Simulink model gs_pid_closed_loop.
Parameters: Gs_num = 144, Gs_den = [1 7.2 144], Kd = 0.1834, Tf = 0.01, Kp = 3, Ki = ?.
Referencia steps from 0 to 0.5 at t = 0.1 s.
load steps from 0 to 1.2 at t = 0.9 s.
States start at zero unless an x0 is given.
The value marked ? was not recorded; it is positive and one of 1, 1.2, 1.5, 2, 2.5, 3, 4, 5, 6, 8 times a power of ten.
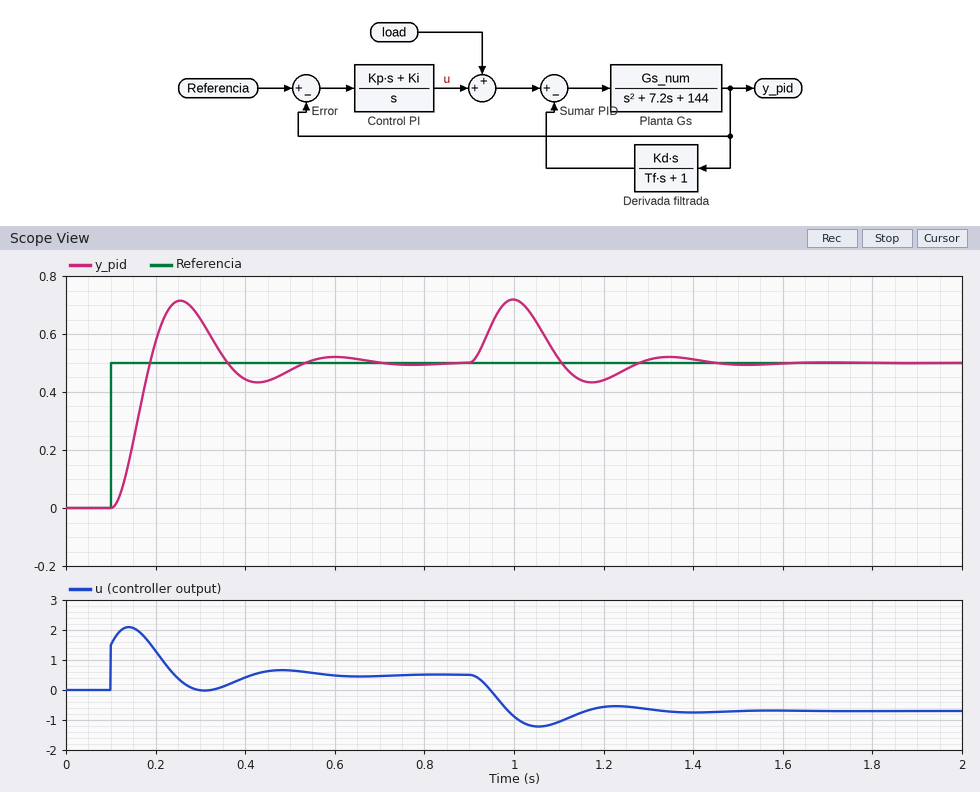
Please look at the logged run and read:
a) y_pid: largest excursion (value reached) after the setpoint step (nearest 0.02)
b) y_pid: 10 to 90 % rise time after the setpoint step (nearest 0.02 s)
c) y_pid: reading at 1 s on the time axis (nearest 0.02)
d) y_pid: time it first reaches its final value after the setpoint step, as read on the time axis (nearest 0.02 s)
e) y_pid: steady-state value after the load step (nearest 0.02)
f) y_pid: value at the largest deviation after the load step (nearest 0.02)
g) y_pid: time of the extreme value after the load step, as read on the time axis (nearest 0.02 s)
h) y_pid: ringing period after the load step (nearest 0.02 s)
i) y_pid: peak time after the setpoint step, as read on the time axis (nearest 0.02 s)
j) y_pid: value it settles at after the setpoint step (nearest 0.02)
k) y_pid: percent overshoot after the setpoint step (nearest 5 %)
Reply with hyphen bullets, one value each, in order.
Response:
- 0.72
- 0.06 s
- 0.72
- 0.18 s
- 0.50
- 0.72
- 1.00 s
- 0.34 s
- 0.26 s
- 0.50
- 45 %
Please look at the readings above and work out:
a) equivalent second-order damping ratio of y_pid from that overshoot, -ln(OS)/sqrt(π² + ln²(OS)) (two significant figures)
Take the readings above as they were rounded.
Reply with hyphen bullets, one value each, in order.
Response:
- 0.25
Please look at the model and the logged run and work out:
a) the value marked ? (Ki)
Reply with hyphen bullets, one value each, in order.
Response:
- 60
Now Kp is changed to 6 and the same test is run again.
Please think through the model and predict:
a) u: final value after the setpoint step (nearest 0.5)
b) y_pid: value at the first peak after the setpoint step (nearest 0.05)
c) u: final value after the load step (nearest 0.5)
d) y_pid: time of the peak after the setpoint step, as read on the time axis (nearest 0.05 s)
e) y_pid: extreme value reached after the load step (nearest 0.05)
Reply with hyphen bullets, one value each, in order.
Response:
- 0.5
- 0.65
- -0.5
- 0.20 s
- 0.65
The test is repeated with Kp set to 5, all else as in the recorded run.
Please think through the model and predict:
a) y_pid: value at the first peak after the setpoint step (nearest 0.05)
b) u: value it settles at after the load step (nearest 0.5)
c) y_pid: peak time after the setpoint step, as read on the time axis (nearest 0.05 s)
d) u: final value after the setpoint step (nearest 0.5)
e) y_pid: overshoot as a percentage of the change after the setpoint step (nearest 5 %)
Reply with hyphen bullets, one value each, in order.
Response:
- 0.65
- -0.5
- 0.20 s
- 0.5
- 30 %
